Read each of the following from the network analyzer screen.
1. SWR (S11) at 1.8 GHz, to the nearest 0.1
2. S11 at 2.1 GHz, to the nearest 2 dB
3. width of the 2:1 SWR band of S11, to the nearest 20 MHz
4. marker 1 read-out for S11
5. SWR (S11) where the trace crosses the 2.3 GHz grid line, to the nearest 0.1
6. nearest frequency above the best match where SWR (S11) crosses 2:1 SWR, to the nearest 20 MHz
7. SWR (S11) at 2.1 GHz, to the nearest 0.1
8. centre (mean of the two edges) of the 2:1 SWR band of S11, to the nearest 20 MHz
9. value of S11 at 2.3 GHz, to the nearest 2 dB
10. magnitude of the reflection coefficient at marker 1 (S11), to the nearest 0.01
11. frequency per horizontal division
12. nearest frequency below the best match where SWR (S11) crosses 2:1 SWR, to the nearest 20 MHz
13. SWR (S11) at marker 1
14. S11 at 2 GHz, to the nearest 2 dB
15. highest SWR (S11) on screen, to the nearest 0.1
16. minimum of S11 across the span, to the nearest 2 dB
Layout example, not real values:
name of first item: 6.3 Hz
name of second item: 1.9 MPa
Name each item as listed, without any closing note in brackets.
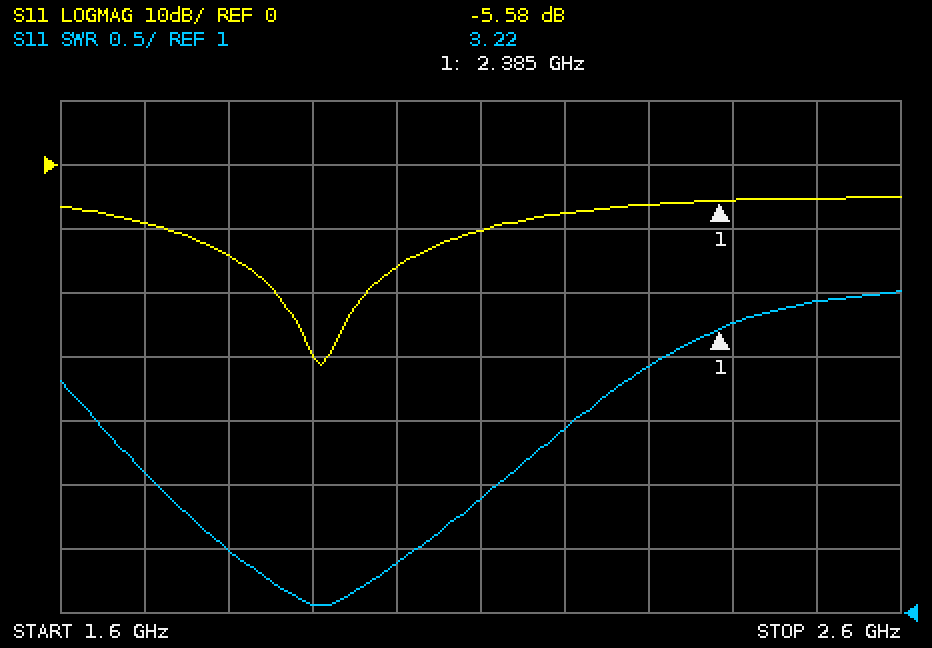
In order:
SWR (S11) at 1.8 GHz, to the nearest 0.1: 1.5
S11 at 2.1 GHz, to the nearest 2 dB: -10 dB
width of the 2:1 SWR band of S11, to the nearest 20 MHz: 400 MHz
marker 1 read-out for S11: -5.58 dB
SWR (S11) where the trace crosses the 2.3 GHz grid line, to the nearest 0.1: 2.9
nearest frequency above the best match where SWR (S11) crosses 2:1 SWR, to the nearest 20 MHz: 2.12 GHz
SWR (S11) at 2.1 GHz, to the nearest 0.1: 1.9
centre (mean of the two edges) of the 2:1 SWR band of S11, to the nearest 20 MHz: 1.92 GHz
value of S11 at 2.3 GHz, to the nearest 2 dB: -6 dB
magnitude of the reflection coefficient at marker 1 (S11), to the nearest 0.01: 0.53
frequency per horizontal division: 100 MHz
nearest frequency below the best match where SWR (S11) crosses 2:1 SWR, to the nearest 20 MHz: 1.72 GHz
SWR (S11) at marker 1: 3.22
S11 at 2 GHz, to the nearest 2 dB: -16 dB
highest SWR (S11) on screen, to the nearest 0.1: 3.5
minimum of S11 across the span, to the nearest 2 dB: -32 dB
